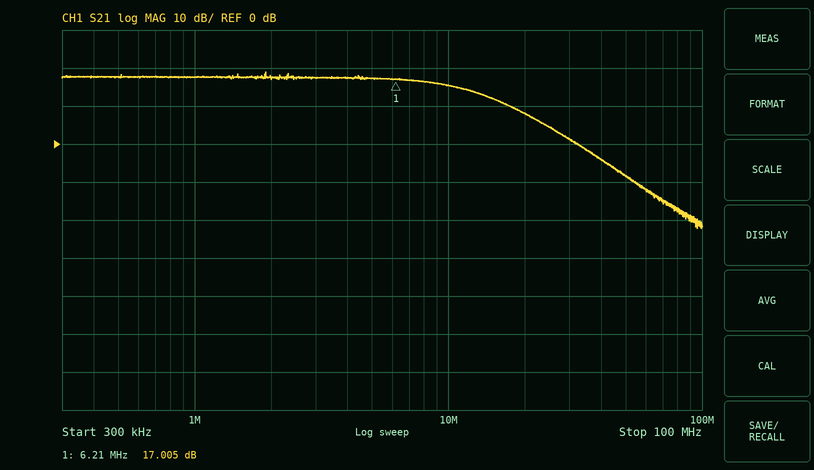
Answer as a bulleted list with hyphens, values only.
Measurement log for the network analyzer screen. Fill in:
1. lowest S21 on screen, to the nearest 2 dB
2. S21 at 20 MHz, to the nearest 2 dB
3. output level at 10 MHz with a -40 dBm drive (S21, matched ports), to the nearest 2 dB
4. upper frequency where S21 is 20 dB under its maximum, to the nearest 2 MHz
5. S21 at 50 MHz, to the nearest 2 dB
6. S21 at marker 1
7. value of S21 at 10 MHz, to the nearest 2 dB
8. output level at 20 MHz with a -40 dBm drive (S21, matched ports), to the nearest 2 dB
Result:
- -22 dB
- 8 dB
- -24 dBm
- 34 MHz
- -8 dB
- 17.005 dB
- 16 dB
- -32 dBm
